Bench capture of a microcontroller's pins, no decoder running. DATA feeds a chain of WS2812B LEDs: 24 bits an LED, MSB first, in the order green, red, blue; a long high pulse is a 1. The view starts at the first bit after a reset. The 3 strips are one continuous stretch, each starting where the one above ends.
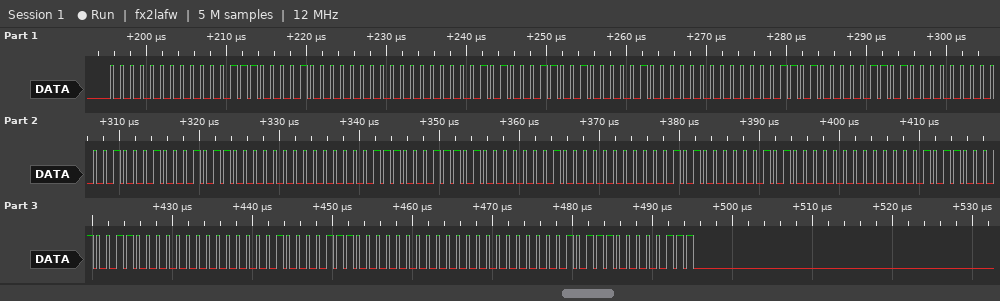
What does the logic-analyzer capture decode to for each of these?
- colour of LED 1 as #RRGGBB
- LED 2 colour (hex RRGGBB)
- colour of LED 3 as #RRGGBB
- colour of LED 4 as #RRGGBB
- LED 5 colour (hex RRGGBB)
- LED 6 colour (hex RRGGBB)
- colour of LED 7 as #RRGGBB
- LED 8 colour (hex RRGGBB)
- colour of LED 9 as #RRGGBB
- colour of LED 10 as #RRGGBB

#0E0010
#050019
#00041A
#000D11
#001607
#011D00
#0A1400
#130B00
#1C0200
#170007
